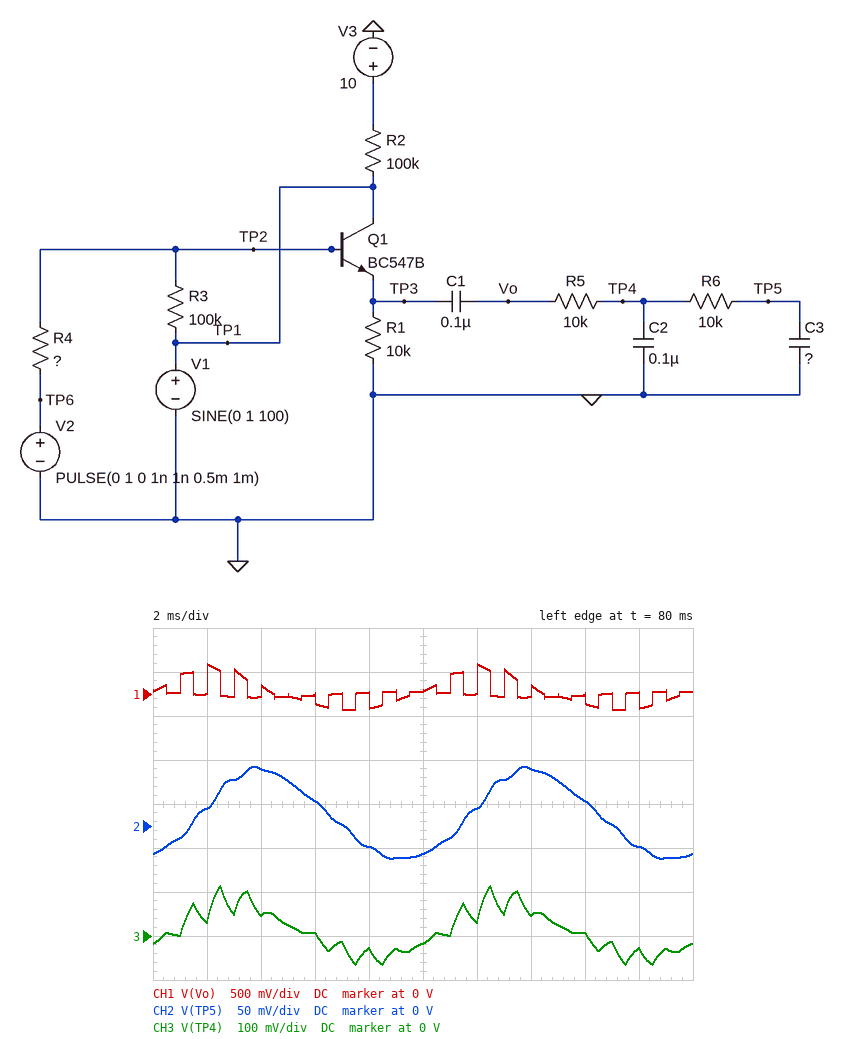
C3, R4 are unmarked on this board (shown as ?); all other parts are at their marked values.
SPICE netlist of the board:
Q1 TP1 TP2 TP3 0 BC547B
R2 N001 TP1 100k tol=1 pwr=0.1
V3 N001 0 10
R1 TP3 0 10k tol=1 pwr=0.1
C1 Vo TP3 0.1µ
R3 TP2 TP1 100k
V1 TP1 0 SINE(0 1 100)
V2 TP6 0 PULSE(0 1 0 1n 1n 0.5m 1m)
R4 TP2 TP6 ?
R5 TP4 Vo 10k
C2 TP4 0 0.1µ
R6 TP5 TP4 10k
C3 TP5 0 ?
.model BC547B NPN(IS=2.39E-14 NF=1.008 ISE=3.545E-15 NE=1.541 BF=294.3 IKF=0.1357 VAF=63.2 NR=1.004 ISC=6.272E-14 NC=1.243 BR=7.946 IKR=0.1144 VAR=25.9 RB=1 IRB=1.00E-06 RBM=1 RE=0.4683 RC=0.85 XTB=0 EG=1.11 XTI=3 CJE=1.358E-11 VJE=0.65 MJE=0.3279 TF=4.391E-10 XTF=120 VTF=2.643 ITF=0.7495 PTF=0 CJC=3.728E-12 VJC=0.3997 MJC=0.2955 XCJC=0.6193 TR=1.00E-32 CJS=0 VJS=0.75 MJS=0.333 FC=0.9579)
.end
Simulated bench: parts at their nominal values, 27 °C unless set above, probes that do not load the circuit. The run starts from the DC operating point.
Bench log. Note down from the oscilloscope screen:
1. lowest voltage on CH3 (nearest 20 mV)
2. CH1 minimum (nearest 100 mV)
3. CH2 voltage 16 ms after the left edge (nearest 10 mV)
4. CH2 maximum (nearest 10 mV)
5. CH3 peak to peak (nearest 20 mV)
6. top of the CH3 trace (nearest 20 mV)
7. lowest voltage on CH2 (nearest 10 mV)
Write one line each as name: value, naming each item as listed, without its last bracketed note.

lowest voltage on CH3: -60 mV
CH1 minimum: -200 mV
CH2 voltage 16 ms after the left edge: 30 mV
CH2 maximum: 70 mV
CH3 peak to peak: 180 mV
top of the CH3 trace: 120 mV
lowest voltage on CH2: -40 mV
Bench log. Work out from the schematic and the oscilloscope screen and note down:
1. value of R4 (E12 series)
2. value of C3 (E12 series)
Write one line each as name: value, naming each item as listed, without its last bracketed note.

value of R4: 120 kΩ
value of C3: 120 nF
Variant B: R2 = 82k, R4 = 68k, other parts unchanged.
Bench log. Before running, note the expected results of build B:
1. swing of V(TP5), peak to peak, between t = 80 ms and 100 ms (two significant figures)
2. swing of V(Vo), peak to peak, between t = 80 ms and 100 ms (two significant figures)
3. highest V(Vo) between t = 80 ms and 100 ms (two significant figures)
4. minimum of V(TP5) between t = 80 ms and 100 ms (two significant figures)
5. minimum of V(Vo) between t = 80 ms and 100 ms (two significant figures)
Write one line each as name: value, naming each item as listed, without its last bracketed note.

swing of V(TP5), peak to peak, between t = 80 ms and 100 ms: 170 mV
swing of V(Vo), peak to peak, between t = 80 ms and 100 ms: 780 mV
highest V(Vo) between t = 80 ms and 100 ms: 350 mV
minimum of V(TP5) between t = 80 ms and 100 ms: -110 mV
minimum of V(Vo) between t = 80 ms and 100 ms: -430 mV
